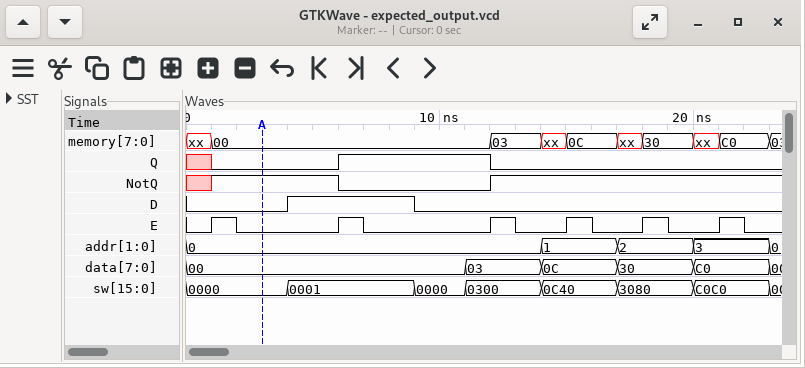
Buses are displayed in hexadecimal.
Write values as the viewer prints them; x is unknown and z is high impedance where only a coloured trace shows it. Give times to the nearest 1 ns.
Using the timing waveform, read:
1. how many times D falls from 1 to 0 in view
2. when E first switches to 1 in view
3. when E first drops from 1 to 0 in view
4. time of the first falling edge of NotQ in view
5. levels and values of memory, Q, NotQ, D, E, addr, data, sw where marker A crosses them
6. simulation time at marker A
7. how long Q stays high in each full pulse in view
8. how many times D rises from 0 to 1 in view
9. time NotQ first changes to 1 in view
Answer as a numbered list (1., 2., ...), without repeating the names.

1. 1
2. 1 ns
3. 2 ns
4. 6 ns
5. memory=00, Q=0, NotQ=1, D=0, E=0, addr=0, data=00, sw=0000
6. 3 ns
7. 6 ns
8. 1
9. 1 ns
